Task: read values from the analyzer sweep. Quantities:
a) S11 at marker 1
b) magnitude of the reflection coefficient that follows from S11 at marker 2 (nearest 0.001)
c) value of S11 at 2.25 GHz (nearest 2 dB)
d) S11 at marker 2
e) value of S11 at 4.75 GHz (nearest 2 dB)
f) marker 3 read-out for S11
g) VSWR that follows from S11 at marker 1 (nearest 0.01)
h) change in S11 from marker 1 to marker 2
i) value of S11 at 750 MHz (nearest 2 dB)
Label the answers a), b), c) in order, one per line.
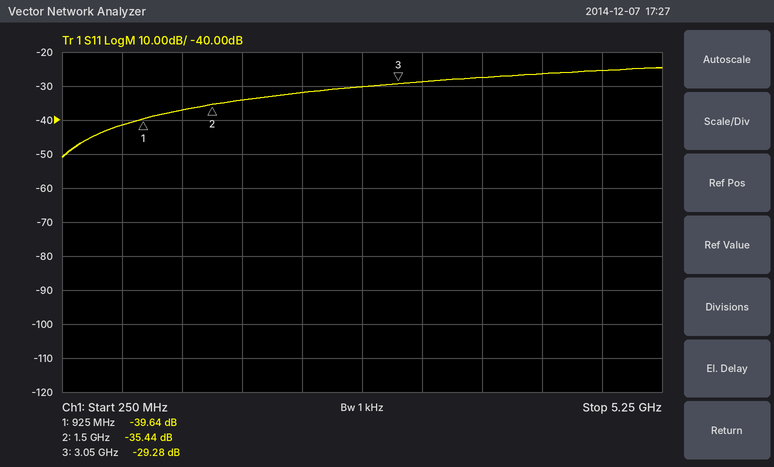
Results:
a) -39.64 dB
b) 0.017
c) -32 dB
d) -35.44 dB
e) -26 dB
f) -29.28 dB
g) 1.02
h) 4.20 dB
i) -42 dB
